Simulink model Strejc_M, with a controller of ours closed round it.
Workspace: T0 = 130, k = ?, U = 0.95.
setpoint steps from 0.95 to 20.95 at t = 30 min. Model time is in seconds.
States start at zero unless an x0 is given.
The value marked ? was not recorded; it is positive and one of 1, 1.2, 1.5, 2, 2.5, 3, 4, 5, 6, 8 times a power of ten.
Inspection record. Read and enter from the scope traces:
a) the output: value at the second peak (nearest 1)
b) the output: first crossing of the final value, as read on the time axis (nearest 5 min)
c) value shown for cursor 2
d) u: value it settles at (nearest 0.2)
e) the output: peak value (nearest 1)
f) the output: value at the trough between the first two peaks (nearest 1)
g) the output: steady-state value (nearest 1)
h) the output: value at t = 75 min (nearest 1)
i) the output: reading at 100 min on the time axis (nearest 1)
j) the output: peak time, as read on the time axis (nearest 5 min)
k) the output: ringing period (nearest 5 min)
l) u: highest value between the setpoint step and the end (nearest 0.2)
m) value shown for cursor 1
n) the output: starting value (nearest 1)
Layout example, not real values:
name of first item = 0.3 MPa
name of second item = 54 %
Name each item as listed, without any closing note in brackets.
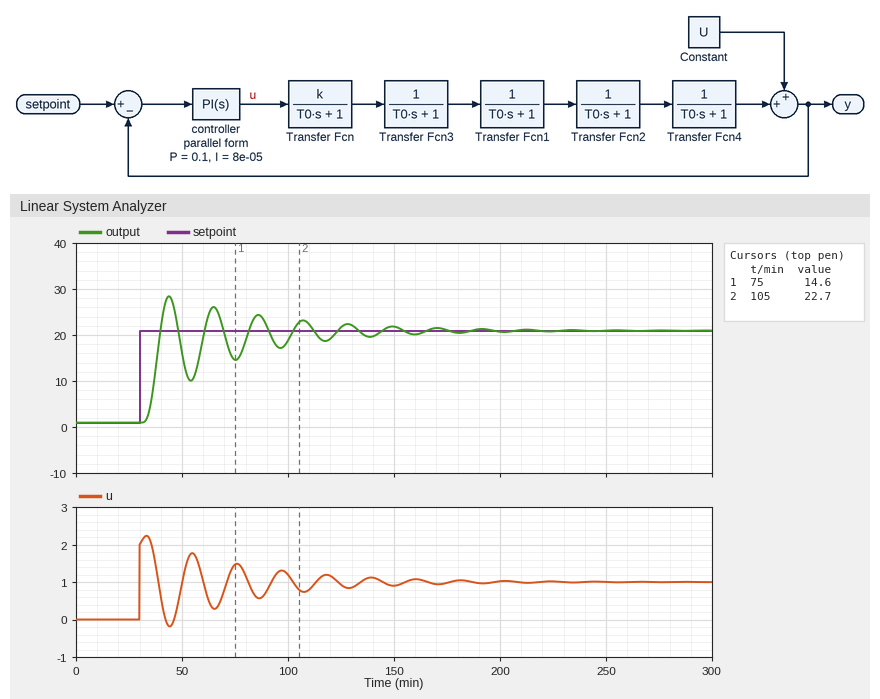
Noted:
the output: value at the second peak = 26
the output: first crossing of the final value, as read on the time axis = 40 min
value shown for cursor 2 = 22.7
u: value it settles at = 1.0
the output: peak value = 28
the output: value at the trough between the first two peaks = 10
the output: steady-state value = 21
the output: value at t = 75 min = 15
the output: reading at 100 min on the time axis = 19
the output: peak time, as read on the time axis = 45 min
the output: ringing period = 20 min
u: highest value between the setpoint step and the end = 2.2
value shown for cursor 1 = 14.6
the output: starting value = 1
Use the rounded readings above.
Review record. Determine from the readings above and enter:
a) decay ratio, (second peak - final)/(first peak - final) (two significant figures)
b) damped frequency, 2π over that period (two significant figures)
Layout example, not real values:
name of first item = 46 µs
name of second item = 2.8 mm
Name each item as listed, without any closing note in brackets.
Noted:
decay ratio, (second peak - final)/(first peak - final) = 0.71
damped frequency, 2π over that period = 0.31 rad/min
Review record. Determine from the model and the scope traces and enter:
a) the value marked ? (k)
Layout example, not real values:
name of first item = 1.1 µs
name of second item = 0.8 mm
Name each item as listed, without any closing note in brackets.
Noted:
the value marked ? = 20
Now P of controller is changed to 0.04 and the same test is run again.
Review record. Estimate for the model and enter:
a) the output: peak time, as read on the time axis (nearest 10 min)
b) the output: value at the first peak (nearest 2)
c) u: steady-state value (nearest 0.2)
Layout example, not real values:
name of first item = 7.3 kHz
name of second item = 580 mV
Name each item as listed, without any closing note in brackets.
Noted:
the output: peak time, as read on the time axis = 50 min
the output: value at the first peak = 22
u: steady-state value = 1.0
